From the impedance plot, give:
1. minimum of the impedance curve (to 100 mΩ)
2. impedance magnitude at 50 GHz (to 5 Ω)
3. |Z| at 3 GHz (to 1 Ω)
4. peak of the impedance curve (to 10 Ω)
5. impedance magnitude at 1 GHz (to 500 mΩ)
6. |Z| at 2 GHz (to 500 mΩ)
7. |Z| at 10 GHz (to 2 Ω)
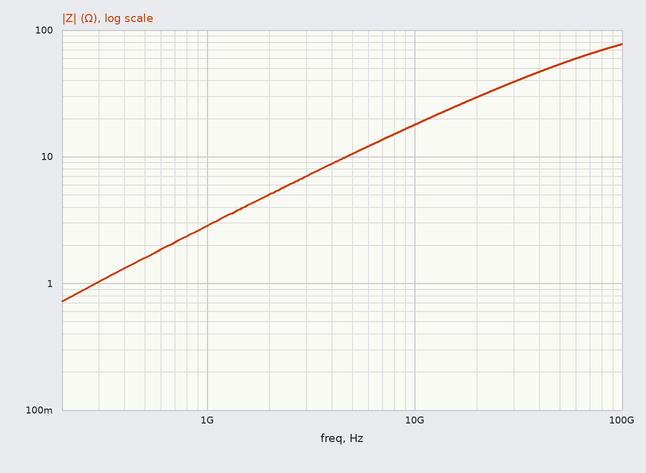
700 mΩ
55 Ω
7 Ω
80 Ω
3.0 Ω
5.0 Ω
18 Ω
